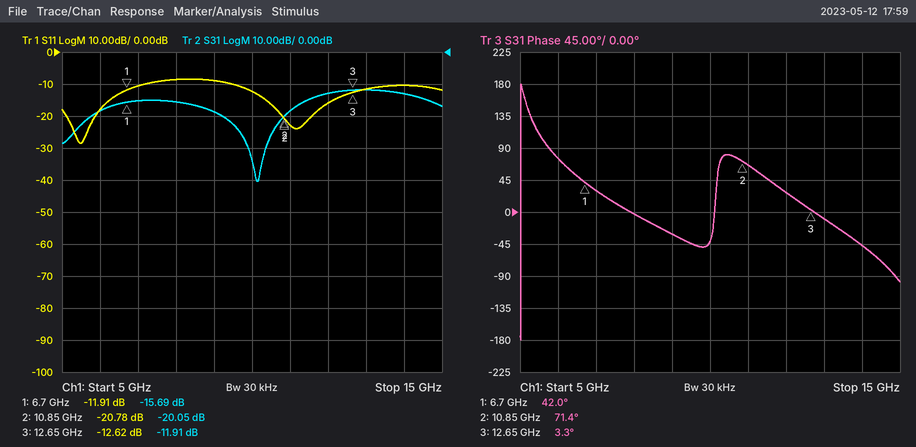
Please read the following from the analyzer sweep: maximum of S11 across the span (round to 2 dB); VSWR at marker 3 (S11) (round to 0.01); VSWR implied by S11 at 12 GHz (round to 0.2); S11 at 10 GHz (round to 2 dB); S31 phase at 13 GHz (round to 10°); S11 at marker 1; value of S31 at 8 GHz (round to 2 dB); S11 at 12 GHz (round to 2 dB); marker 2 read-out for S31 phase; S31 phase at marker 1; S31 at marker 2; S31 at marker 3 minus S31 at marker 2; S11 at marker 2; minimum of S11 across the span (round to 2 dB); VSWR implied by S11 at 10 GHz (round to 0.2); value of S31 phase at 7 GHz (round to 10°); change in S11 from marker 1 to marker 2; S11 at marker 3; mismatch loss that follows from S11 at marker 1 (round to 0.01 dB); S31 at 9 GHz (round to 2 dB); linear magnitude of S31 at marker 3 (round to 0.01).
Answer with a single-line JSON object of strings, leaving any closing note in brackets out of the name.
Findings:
{"maximum of S11 across the span": "-8 dB", "VSWR at marker 3 (S11)": "1.61", "VSWR implied by S11 at 12 GHz": "1.4", "S11 at 10 GHz": "-12 dB", "S31 phase at 13 GHz": "-10°", "S11 at marker 1": "-11.91 dB", "value of S31 at 8 GHz": "-16 dB", "S11 at 12 GHz": "-16 dB", "marker 2 read-out for S31 phase": "71.4°", "S31 phase at marker 1": "42.0°", "S31 at marker 2": "-20.05 dB", "S31 at marker 3 minus S31 at marker 2": "8.14 dB", "S11 at marker 2": "-20.78 dB", "minimum of S11 across the span": "-28 dB", "VSWR implied by S11 at 10 GHz": "1.6", "value of S31 phase at 7 GHz": "30°", "change in S11 from marker 1 to marker 2": "-8.87 dB", "S11 at marker 3": "-12.62 dB", "mismatch loss that follows from S11 at marker 1": "0.29 dB", "S31 at 9 GHz": "-18 dB", "linear magnitude of S31 at marker 3": "0.25"}
